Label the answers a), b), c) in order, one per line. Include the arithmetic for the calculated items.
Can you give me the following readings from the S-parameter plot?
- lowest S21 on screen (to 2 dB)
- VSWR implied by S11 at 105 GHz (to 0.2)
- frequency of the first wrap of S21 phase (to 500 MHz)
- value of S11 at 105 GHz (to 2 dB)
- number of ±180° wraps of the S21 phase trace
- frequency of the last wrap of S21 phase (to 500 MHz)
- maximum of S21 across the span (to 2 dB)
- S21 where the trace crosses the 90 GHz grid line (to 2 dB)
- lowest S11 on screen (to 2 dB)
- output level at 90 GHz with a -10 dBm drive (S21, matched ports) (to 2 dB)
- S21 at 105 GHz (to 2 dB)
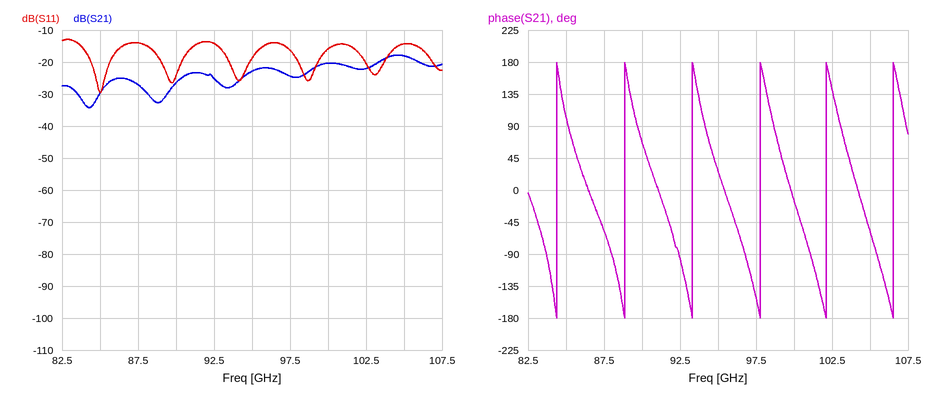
a) -34 dB
b) |Γ| = 10^(-14/20) = 0.1995; VSWR = (1 + 0.1995)/(1 − 0.1995) ≈ 1.50, so 1.4 to the nearest 0.2
c) 84.5 GHz
d) -14 dB
e) 6
f) 106.5 GHz
g) -18 dB
h) -26 dB
i) -30 dB
j) -10 dBm + (-26 dB) = -36 dBm
k) -18 dB
